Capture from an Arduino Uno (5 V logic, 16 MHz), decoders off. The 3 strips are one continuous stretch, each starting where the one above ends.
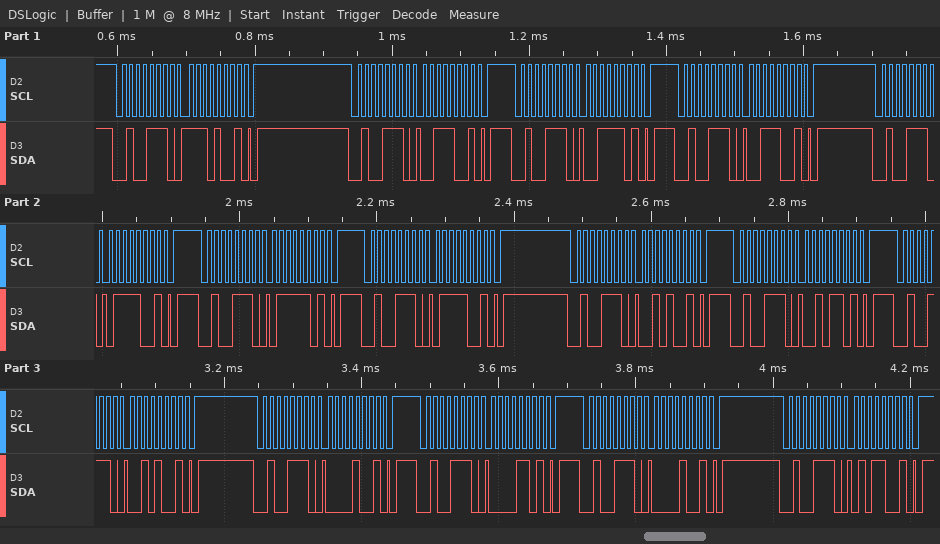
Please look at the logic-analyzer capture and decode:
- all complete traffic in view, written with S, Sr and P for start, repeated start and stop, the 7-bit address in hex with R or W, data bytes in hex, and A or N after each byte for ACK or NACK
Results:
S 27W A E9 A P S 27W A 39 A P S 27W A 3D A P S 27W A 39 A P S 27W A 79 A P S 27W A 7D A P S 27W A 79 A P S 27W A 29 A P S 27W A 2D A P S 27W A 29 A P S 27W A 09 A P S 27W A 0D A P S 27W A 09 A P S 27W A 59 A P
